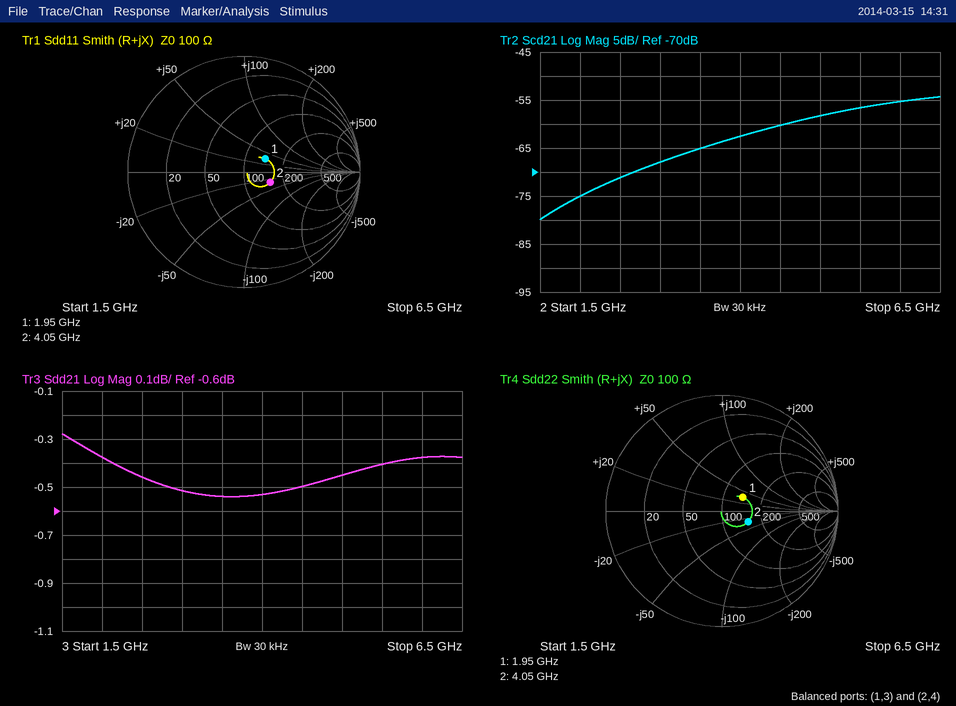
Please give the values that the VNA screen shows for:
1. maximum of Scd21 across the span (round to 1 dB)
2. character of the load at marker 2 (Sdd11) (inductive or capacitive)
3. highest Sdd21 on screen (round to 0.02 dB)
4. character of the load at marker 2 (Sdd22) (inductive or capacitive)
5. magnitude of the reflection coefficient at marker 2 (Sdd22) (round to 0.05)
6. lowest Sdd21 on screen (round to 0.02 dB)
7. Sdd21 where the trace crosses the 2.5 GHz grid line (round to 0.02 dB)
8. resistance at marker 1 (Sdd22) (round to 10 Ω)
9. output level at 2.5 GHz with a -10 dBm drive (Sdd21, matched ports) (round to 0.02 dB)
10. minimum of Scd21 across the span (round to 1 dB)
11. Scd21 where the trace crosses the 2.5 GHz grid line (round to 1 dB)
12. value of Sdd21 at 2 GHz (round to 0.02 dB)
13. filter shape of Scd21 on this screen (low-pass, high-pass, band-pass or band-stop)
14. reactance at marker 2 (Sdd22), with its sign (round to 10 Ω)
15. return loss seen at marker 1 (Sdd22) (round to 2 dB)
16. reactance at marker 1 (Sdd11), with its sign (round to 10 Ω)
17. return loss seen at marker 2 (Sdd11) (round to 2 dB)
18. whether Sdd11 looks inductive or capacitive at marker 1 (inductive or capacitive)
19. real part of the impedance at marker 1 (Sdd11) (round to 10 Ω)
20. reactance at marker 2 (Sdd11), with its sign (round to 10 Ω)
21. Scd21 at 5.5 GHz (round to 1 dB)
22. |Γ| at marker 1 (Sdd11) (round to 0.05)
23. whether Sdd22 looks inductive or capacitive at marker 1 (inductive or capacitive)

-54 dB
capacitive
-0.28 dB
capacitive
0.25
-0.54 dB
-0.46 dB
140 Ω
-10.46 dBm
-80 dB
-71 dB
-0.38 dB
high-pass
-30 Ω
14 dB
+30 Ω
12 dB
inductive
140 Ω
-30 Ω
-57 dB
0.20
inductive
